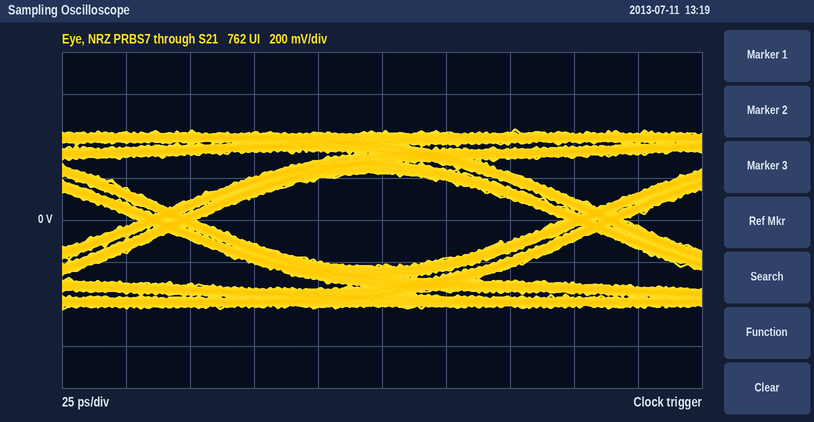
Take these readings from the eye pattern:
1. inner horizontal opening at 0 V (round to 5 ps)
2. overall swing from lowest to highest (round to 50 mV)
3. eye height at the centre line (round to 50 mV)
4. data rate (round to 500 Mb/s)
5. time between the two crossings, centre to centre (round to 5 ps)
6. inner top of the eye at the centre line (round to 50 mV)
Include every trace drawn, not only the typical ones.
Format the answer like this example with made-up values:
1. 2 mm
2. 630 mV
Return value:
1. 145 ps
2. 850 mV
3. 450 mV
4. 6.0 Gb/s
5. 165 ps
6. 200 mV
